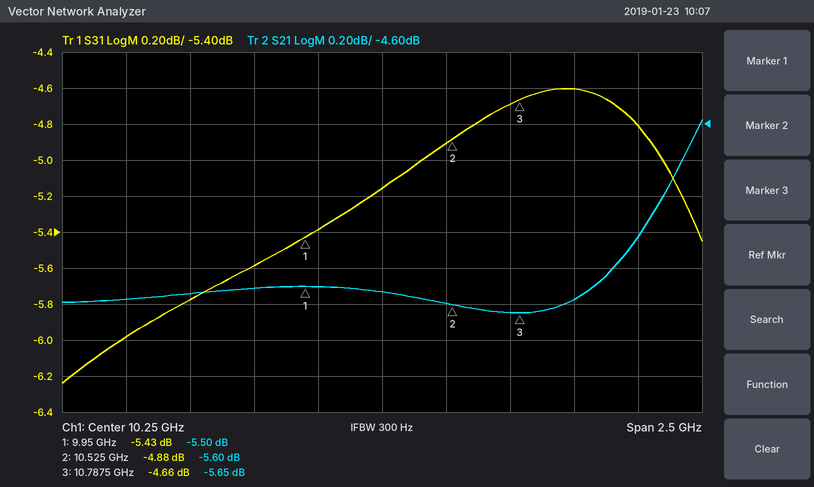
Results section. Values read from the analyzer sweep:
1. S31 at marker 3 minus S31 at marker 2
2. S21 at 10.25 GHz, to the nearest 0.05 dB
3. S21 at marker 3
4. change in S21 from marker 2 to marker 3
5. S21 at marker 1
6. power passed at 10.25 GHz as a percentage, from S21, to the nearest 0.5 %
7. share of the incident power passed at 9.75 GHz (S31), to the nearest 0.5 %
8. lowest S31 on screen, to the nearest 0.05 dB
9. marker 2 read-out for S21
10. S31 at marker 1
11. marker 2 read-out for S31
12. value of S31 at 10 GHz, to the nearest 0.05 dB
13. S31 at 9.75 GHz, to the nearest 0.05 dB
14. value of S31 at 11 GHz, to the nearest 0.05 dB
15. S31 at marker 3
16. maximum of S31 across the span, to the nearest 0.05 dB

0.22 dB
-5.55 dB
-5.65 dB
-0.05 dB
-5.50 dB
28.0 %
27.5 %
-6.25 dB
-5.60 dB
-5.43 dB
-4.88 dB
-5.40 dB
-5.60 dB
-4.60 dB
-4.66 dB
-4.60 dB
